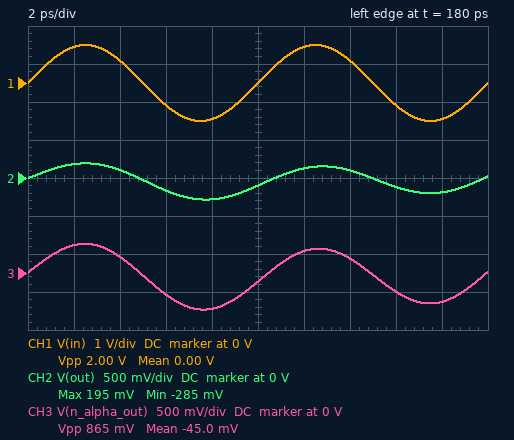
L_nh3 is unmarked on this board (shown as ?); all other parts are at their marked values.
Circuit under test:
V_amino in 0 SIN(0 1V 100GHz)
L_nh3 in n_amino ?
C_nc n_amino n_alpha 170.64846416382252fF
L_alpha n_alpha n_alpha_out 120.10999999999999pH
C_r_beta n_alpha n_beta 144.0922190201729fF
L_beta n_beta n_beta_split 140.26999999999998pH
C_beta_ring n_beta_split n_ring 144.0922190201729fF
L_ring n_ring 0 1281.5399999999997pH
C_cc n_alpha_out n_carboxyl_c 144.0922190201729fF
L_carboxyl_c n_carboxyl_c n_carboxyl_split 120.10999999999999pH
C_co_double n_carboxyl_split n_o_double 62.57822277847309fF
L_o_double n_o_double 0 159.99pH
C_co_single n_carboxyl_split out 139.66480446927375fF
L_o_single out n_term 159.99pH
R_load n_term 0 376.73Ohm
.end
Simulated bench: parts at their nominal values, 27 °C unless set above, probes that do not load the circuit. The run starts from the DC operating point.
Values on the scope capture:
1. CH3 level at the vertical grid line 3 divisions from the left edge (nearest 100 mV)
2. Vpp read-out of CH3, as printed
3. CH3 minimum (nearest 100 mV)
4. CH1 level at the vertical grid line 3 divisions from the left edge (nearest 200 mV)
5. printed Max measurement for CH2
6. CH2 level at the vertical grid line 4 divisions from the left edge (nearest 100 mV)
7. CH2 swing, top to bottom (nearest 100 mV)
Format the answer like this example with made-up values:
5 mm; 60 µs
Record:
-300 mV; 865 mV; -500 mV; -600 mV; 195 mV; -300 mV; 500 mV
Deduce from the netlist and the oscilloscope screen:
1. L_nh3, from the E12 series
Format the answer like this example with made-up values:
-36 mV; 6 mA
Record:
180 pH
